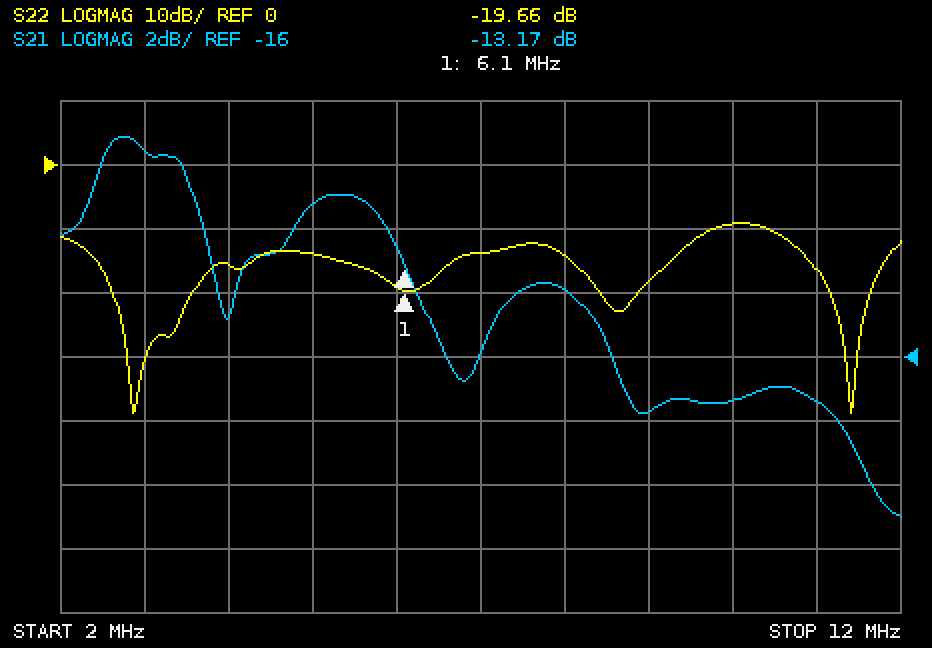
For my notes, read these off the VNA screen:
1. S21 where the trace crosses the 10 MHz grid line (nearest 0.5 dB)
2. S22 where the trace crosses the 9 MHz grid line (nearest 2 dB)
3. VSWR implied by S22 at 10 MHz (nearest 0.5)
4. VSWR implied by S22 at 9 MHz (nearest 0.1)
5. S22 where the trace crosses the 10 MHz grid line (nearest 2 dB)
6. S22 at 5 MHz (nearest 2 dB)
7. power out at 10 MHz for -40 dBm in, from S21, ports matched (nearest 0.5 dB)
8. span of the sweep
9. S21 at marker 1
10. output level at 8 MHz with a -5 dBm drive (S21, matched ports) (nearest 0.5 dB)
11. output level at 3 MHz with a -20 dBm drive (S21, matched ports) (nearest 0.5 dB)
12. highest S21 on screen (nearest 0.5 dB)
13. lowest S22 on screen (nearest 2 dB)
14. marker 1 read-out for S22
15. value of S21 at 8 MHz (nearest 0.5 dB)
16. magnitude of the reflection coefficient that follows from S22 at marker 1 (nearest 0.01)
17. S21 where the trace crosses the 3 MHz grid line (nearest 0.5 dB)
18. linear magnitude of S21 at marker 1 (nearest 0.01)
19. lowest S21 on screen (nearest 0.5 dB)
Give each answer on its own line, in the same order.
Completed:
-17.5 dB
-18 dB
2.0
1.3
-10 dB
-14 dB
-57.5 dBm
10 MHz
-13.17 dB
-19.0 dBm
-29.5 dBm
-9.0 dB
-38 dB
-19.66 dB
-14.0 dB
0.10
-9.5 dB
0.22
-21.0 dB
